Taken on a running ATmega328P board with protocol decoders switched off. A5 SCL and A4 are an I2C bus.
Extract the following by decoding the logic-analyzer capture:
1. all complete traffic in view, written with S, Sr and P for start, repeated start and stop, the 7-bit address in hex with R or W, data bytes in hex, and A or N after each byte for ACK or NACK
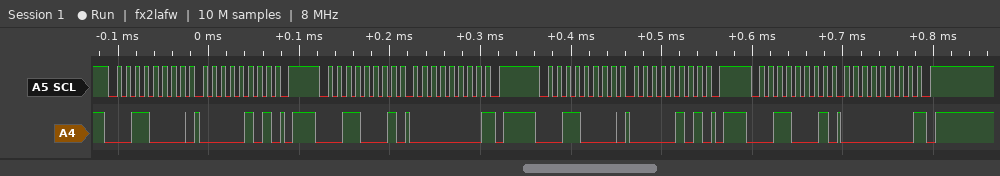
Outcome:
S 18W A 05 A P S 18R A 00 N P S 18W A 05 A P S 18R A 00 N P
